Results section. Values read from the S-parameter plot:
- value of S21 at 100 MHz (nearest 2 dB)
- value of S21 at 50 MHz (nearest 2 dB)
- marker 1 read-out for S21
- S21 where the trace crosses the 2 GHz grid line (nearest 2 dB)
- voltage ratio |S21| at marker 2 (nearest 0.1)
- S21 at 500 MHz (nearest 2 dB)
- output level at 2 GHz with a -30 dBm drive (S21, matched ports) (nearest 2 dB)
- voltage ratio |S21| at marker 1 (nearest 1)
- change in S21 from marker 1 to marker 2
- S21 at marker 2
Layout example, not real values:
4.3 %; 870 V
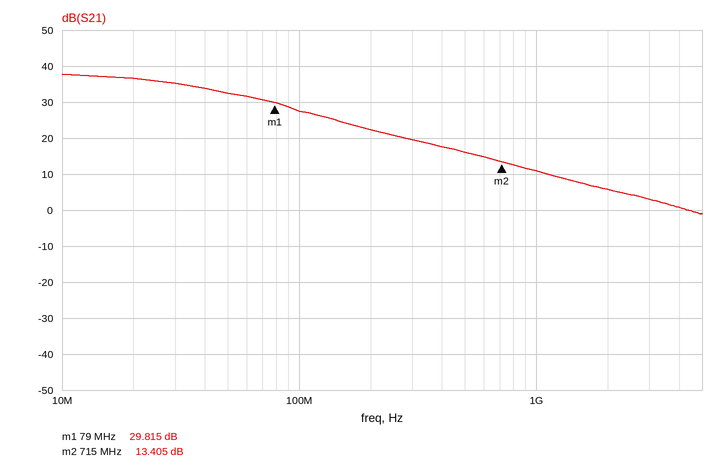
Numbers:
28 dB; 32 dB; 29.815 dB; 6 dB; 4.7; 16 dB; -24 dBm; 31; -16.410 dB; 13.405 dB
